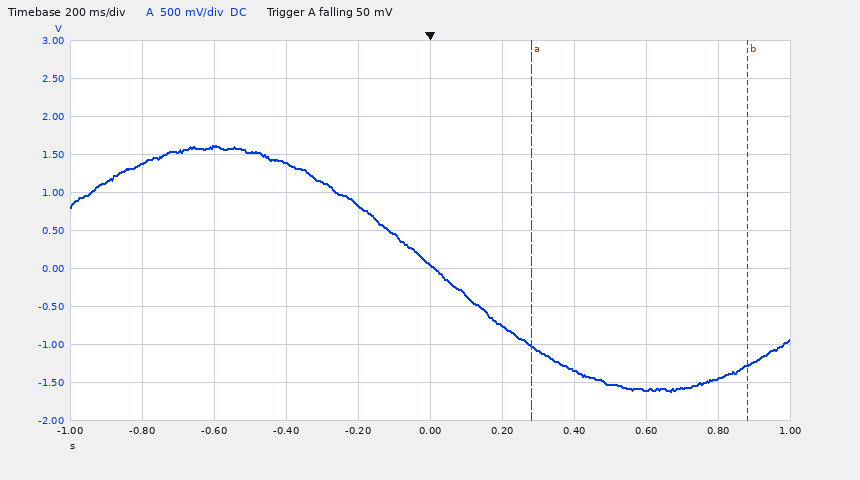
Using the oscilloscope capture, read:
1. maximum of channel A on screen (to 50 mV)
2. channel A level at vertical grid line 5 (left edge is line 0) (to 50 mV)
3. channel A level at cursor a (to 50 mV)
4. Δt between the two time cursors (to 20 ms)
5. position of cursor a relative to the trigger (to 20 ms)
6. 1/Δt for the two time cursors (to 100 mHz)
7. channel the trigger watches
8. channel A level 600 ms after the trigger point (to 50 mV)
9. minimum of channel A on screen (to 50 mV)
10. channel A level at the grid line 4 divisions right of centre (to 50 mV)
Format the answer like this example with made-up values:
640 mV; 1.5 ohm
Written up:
1.60 V; 50 mV; -1.00 V; 600 ms; +280 ms; 1.7 Hz; channel A; -1.60 V; -1.60 V; -1.45 V
